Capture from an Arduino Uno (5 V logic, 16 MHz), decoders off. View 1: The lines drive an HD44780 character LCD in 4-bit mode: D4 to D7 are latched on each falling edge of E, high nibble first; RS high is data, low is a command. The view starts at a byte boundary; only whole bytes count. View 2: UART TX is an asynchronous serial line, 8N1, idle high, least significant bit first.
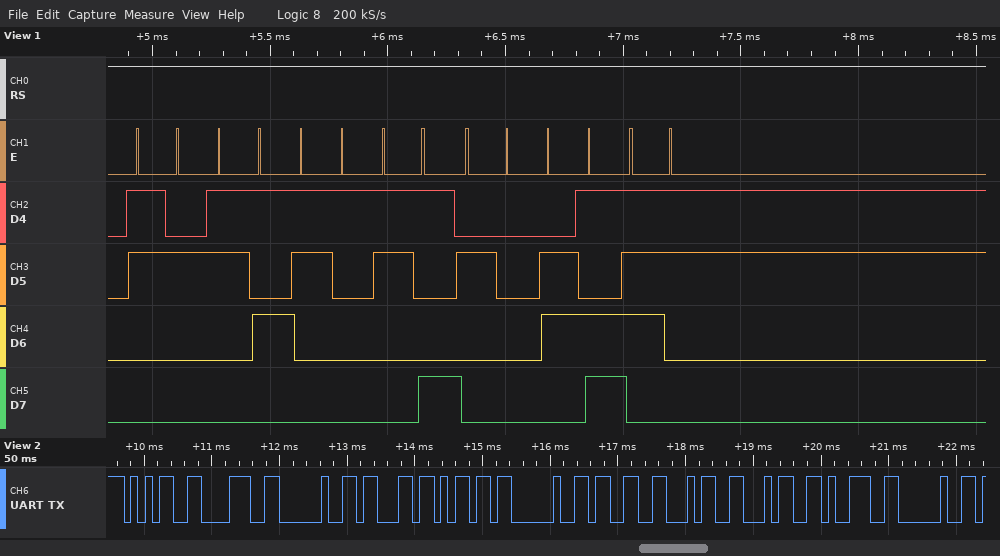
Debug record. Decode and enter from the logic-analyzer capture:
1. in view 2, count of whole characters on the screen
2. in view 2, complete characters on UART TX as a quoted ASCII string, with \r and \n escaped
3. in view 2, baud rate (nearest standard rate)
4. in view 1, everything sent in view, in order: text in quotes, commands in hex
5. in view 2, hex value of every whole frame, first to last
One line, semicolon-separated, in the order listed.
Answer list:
11; "58 cm 3449 "; 9600 baud; "2519 ms"; 35 38 20 63 6D 20 33 34 34 39 20
